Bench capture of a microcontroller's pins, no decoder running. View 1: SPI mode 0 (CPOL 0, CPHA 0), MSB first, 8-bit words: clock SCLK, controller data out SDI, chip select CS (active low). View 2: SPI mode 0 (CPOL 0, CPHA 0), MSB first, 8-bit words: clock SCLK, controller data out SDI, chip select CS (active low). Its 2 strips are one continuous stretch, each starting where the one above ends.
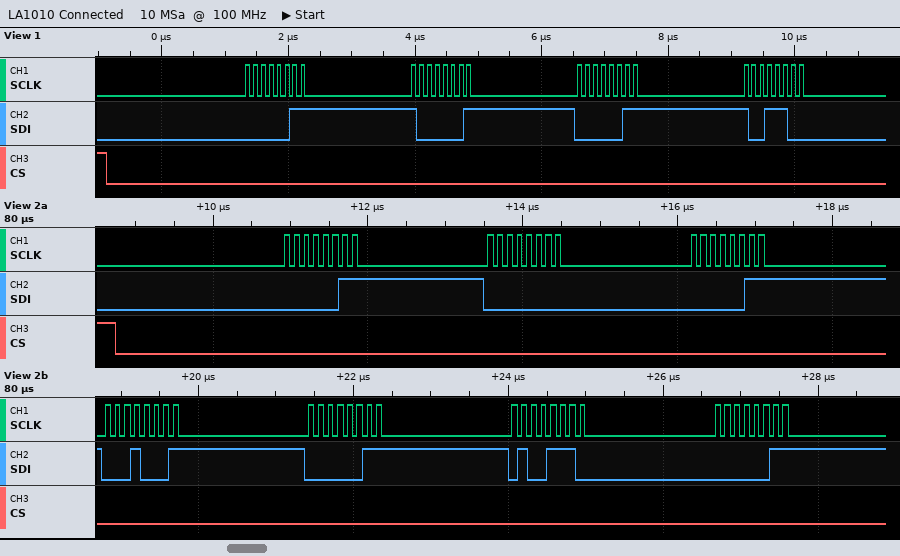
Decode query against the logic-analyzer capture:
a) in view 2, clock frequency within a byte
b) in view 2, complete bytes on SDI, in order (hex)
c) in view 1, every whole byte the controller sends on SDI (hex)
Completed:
8 MHz
03 00 03 11 03 4E 03
0x03 0x81 0x03 0x9C
